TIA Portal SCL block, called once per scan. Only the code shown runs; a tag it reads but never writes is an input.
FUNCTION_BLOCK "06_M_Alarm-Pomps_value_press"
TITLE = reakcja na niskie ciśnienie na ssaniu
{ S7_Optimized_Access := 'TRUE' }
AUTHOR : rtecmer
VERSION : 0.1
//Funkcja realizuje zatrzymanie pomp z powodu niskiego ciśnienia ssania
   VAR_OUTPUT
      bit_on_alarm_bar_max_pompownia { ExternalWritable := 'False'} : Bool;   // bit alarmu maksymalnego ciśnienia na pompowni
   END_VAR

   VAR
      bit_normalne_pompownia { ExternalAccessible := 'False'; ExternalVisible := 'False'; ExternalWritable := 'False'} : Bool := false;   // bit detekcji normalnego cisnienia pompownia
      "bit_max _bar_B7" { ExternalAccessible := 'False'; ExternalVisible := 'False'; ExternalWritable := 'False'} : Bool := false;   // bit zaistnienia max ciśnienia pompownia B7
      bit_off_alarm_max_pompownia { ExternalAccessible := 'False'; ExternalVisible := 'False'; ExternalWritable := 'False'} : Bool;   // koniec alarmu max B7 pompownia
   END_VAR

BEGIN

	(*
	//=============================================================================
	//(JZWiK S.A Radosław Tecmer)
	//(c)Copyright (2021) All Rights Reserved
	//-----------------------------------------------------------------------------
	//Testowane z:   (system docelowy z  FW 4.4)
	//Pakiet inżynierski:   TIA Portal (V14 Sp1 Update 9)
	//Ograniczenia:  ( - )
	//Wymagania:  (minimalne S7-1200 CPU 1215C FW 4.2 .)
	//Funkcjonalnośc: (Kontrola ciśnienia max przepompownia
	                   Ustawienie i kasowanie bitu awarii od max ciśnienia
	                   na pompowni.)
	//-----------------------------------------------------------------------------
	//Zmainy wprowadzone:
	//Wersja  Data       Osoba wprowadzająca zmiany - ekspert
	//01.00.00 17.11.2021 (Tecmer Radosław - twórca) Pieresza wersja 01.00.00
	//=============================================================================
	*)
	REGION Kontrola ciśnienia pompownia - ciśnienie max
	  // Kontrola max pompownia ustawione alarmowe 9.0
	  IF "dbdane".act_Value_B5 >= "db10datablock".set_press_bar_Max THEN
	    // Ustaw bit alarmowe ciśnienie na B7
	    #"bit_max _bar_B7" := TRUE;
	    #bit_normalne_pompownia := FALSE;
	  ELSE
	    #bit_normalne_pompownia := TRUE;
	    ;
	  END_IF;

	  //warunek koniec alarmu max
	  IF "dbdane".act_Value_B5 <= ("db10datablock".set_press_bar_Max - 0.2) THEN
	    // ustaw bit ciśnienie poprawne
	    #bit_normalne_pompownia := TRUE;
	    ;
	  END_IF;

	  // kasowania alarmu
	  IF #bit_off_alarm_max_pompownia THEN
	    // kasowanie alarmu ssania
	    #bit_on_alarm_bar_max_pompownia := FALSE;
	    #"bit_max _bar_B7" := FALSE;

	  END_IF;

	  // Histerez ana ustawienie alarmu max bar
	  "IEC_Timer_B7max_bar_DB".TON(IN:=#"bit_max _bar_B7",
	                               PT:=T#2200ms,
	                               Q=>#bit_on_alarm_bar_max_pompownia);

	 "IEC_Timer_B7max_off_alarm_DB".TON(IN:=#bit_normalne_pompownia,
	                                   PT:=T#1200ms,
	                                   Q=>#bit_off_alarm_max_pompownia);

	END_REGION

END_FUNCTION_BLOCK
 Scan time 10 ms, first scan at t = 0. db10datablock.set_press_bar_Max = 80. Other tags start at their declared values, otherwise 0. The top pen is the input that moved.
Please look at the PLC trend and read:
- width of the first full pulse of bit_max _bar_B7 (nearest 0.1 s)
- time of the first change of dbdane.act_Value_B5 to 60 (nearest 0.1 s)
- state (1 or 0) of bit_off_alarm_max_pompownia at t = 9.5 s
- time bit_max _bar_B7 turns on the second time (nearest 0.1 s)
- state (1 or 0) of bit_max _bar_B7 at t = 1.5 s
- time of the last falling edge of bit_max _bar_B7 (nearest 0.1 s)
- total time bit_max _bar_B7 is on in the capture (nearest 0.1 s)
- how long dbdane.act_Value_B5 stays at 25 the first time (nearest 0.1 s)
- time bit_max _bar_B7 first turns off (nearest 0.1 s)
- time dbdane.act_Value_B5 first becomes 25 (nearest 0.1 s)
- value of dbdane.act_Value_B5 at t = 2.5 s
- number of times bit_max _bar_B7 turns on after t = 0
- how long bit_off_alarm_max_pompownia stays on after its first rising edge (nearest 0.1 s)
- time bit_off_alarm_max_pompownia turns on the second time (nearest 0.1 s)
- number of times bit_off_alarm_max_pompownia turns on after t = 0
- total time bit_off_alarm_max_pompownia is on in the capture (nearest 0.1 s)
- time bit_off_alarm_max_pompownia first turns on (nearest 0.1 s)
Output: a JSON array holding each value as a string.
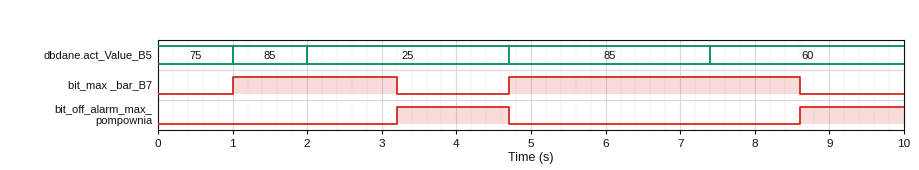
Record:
["2.2 s", "7.4 s", "1", "4.7 s", "1", "8.6 s", "6.1 s", "2.7 s", "3.2 s", "2.0 s", "25", "2", "1.5 s", "8.6 s", "2", "2.9 s", "3.2 s"]
